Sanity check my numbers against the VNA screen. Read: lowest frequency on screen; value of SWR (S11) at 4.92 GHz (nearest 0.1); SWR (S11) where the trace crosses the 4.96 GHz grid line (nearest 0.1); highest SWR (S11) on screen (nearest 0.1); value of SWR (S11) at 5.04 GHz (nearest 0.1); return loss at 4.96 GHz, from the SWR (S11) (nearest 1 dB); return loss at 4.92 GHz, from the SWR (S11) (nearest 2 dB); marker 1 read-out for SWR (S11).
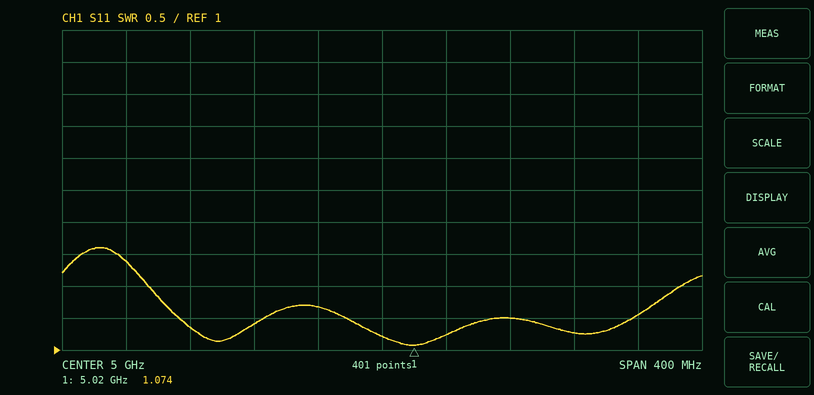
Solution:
4.8 GHz
1.4
1.7
2.6
1.2
12 dB
16 dB
1.074
